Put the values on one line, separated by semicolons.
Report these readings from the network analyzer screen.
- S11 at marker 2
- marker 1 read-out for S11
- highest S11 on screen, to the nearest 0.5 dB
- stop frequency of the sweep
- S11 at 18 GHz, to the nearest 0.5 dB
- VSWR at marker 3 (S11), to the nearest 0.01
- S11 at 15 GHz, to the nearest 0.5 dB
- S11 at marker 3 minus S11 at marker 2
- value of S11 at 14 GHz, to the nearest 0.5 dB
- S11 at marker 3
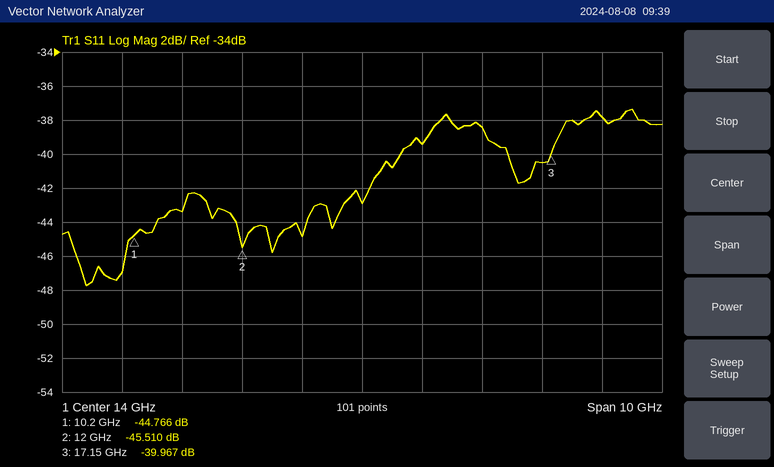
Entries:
-45.510 dB; -44.766 dB; -37.5 dB; 19 GHz; -38.0 dB; 1.02; -39.5 dB; 5.543 dB; -43.0 dB; -39.967 dB
